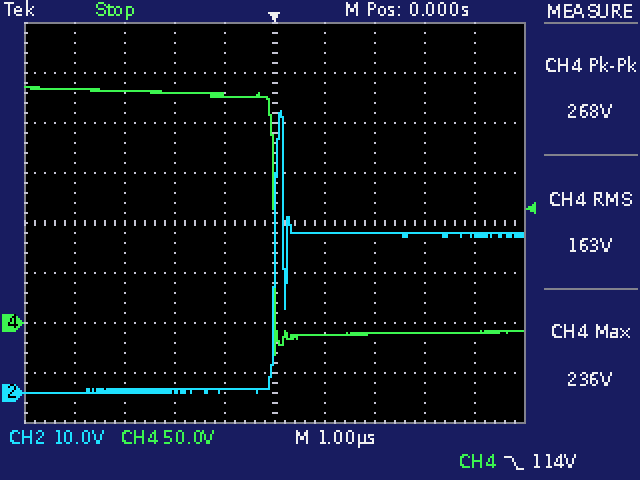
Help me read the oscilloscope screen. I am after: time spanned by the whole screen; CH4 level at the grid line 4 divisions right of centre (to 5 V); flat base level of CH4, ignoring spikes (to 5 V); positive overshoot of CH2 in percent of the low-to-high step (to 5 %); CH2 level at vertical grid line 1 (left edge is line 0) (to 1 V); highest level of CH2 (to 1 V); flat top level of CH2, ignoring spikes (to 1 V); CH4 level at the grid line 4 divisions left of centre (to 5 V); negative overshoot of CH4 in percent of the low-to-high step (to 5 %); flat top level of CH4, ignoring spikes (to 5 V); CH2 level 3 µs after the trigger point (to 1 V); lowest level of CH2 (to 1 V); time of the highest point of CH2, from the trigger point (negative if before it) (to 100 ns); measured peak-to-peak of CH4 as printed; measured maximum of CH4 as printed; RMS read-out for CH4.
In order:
10 µs
-10 V
-10 V
80 %
0 V
56 V
32 V
235 V
10 %
230 V
32 V
0 V
+100 ns
268 V
236 V
163 V
